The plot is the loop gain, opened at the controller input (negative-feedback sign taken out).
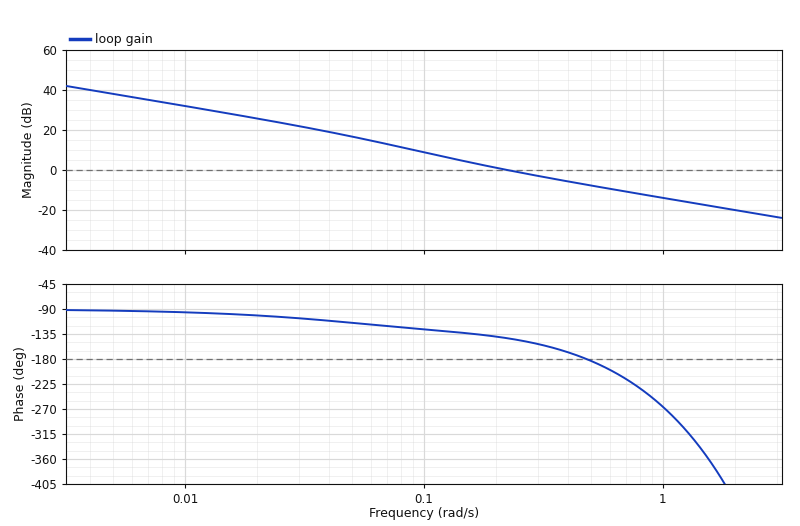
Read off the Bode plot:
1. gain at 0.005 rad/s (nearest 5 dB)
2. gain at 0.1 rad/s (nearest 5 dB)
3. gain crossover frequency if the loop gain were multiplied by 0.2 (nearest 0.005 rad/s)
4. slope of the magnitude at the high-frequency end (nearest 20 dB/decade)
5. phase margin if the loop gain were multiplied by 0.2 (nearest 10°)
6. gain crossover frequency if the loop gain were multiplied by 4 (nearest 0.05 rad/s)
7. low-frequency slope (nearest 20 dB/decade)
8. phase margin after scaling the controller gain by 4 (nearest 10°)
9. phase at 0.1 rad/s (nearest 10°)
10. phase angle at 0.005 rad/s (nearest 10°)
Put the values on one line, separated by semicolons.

40 dB; 10 dB; 0.065 rad/s; -20 dB/decade; 60°; 0.80 rad/s; -20 dB/decade; -50°; -130°; -90°
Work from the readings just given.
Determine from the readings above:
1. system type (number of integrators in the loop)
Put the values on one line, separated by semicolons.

1
